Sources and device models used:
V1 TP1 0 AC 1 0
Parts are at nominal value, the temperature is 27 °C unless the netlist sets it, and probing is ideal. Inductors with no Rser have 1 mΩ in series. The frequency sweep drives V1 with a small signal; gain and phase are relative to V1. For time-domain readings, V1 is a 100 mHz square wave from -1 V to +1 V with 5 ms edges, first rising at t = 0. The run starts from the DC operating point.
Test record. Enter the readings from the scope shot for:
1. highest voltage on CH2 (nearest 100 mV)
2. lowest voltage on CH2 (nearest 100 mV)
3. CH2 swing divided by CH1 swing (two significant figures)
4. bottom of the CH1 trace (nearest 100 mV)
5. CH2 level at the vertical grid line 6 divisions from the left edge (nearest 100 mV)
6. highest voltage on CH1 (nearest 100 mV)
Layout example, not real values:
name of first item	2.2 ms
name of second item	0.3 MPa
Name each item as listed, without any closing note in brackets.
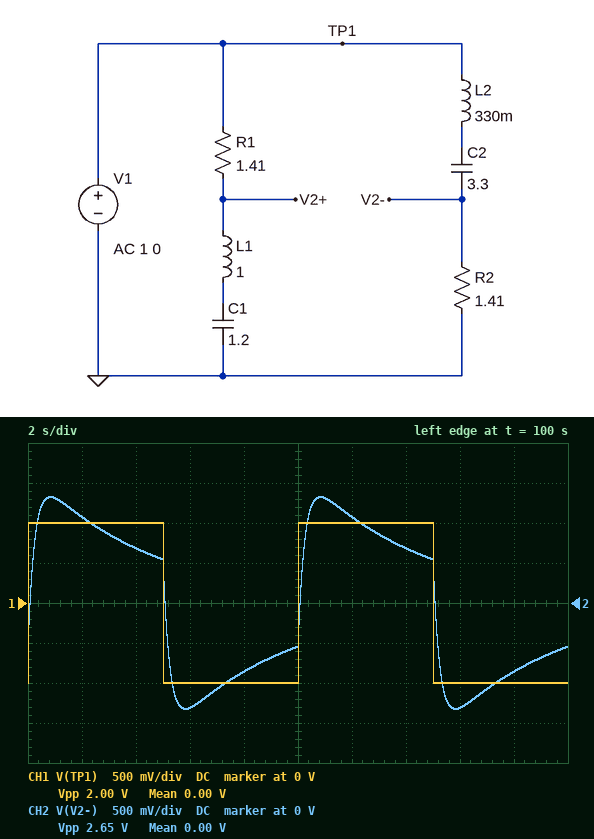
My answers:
highest voltage on CH2	1.3 V
lowest voltage on CH2	-1.3 V
CH2 swing divided by CH1 swing	1.3
bottom of the CH1 trace	-1.0 V
CH2 level at the vertical grid line 6 divisions from the left edge	1.1 V
highest voltage on CH1	1.0 V
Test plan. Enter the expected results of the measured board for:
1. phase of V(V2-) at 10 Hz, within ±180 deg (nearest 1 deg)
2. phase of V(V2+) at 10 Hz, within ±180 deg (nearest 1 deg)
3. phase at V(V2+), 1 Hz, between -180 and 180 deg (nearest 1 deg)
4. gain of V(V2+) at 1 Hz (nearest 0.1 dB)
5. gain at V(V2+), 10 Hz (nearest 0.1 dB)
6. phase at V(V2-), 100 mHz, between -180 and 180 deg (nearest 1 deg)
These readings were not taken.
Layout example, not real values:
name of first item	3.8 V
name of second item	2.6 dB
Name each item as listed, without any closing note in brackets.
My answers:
phase of V(V2-) at 10 Hz, within ±180 deg	-86 deg
phase of V(V2+) at 10 Hz, within ±180 deg	1 deg
phase at V(V2+), 1 Hz, between -180 and 180 deg	13 deg
gain of V(V2+) at 1 Hz	-0.2 dB
gain at V(V2+), 10 Hz	0 dB
phase at V(V2-), 100 mHz, between -180 and 180 deg	11 deg
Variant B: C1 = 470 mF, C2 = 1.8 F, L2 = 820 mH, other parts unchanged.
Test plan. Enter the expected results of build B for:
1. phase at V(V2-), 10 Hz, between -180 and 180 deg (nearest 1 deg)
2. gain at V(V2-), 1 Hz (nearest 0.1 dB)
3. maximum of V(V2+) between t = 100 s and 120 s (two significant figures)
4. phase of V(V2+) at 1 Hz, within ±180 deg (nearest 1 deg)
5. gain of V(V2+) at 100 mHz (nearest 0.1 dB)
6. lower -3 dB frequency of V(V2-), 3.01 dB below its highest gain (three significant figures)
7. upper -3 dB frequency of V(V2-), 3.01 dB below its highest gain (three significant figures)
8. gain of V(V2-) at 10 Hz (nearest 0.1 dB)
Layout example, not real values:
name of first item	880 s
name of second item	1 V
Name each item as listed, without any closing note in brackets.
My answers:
phase at V(V2-), 10 Hz, between -180 and 180 deg	-88 deg
gain at V(V2-), 1 Hz	-11.4 dB
maximum of V(V2+) between t = 100 s and 120 s	1.2 V
phase of V(V2+) at 1 Hz, within ±180 deg	13 deg
gain of V(V2+) at 100 mHz	-1.0 dB
lower -3 dB frequency of V(V2-), 3.01 dB below its highest gain	52.6 mHz
upper -3 dB frequency of V(V2-), 3.01 dB below its highest gain	326 mHz
gain of V(V2-) at 10 Hz	-31.3 dB
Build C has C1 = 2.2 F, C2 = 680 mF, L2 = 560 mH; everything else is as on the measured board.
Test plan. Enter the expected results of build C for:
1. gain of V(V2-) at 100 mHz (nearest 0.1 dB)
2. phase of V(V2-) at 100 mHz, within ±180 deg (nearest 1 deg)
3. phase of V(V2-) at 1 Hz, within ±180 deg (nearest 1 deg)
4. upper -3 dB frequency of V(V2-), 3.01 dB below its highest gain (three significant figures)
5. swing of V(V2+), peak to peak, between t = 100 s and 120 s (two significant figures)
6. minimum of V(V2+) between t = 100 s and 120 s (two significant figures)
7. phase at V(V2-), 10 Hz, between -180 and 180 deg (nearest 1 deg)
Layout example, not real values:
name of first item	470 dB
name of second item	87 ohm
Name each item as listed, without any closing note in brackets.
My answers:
gain of V(V2-) at 100 mHz	-4.8 dB
phase of V(V2-) at 100 mHz, within ±180 deg	55 deg
phase of V(V2-) at 1 Hz, within ±180 deg	-67 deg
upper -3 dB frequency of V(V2-), 3.01 dB below its highest gain	527 mHz
swing of V(V2+), peak to peak, between t = 100 s and 120 s	2.9 V
minimum of V(V2+) between t = 100 s and 120 s	-1.4 V
phase at V(V2-), 10 Hz, between -180 and 180 deg	-88 deg
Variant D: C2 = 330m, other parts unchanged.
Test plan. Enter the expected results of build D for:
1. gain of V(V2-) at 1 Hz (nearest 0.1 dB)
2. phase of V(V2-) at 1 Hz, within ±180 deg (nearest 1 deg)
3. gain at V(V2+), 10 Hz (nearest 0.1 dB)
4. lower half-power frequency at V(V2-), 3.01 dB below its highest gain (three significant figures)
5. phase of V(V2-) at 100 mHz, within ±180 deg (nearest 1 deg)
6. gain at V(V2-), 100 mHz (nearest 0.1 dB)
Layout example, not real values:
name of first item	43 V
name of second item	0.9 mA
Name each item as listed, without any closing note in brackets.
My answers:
gain of V(V2-) at 1 Hz	-3.6 dB
phase of V(V2-) at 1 Hz, within ±180 deg	-48 deg
gain at V(V2+), 10 Hz	0 dB
lower half-power frequency at V(V2-), 3.01 dB below its highest gain	250 mHz
phase of V(V2-) at 100 mHz, within ±180 deg	73 deg
gain at V(V2-), 100 mHz	-10.7 dB
